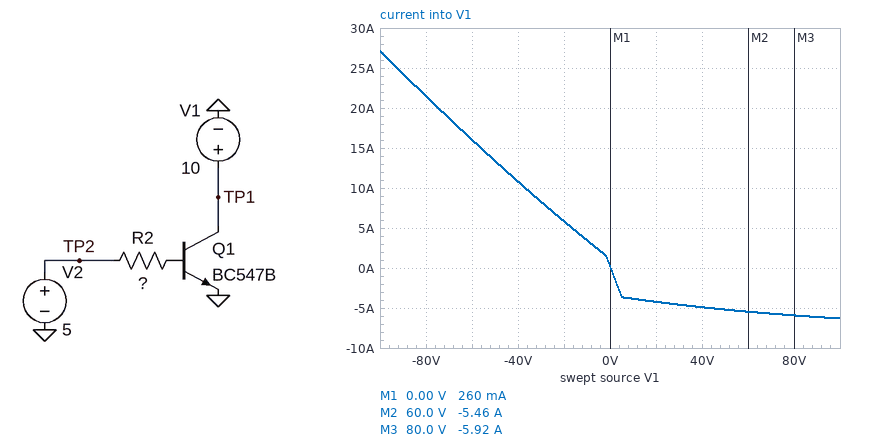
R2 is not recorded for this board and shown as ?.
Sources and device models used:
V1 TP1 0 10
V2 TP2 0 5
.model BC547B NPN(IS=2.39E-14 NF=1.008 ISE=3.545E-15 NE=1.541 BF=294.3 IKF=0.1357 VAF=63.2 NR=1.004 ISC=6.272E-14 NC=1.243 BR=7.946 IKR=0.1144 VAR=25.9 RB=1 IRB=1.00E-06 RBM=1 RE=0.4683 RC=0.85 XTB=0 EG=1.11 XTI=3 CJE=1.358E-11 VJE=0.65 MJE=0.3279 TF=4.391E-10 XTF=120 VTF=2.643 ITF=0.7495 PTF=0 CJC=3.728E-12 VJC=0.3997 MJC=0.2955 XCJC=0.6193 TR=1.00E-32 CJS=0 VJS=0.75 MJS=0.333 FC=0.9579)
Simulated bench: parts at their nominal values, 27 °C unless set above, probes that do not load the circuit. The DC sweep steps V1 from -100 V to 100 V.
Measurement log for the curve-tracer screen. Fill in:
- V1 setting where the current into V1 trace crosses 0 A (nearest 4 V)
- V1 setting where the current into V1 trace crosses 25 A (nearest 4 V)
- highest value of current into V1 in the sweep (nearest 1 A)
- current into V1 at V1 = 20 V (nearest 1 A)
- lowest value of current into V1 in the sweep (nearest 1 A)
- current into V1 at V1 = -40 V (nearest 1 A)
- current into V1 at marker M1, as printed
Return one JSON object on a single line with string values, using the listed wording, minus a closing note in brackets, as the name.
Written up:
{"V1 setting where the current into V1 trace crosses 0 A": "0 V", "V1 setting where the current into V1 trace crosses 25 A": "-92 V", "highest value of current into V1 in the sweep": "27 A", "current into V1 at V1 = 20 V": "-4 A", "lowest value of current into V1 in the sweep": "-6 A", "current into V1 at V1 = -40 V": "11 A", "current into V1 at marker M1, as printed": "260 mA"}
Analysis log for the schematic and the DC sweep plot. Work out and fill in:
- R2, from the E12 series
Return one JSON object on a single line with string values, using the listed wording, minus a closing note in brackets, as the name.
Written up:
{"R2, from the E12 series": "4.7 Ω"}
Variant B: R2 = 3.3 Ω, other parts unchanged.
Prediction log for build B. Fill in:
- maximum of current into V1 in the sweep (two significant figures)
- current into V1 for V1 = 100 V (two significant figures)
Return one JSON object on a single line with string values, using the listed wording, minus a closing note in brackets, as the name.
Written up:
{"maximum of current into V1 in the sweep": "32 A", "current into V1 for V1 = 100 V": "-6.6 A"}
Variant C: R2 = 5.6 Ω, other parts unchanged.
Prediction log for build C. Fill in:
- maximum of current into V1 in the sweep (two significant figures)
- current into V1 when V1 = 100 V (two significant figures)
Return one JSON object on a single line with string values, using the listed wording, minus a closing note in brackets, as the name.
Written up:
{"maximum of current into V1 in the sweep": "25 A", "current into V1 when V1 = 100 V": "-6.1 A"}
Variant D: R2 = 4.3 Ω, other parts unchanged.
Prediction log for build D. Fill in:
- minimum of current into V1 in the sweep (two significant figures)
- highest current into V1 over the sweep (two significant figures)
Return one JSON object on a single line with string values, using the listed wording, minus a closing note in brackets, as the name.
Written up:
{"minimum of current into V1 in the sweep": "-6.4 A", "highest current into V1 over the sweep": "28 A"}
